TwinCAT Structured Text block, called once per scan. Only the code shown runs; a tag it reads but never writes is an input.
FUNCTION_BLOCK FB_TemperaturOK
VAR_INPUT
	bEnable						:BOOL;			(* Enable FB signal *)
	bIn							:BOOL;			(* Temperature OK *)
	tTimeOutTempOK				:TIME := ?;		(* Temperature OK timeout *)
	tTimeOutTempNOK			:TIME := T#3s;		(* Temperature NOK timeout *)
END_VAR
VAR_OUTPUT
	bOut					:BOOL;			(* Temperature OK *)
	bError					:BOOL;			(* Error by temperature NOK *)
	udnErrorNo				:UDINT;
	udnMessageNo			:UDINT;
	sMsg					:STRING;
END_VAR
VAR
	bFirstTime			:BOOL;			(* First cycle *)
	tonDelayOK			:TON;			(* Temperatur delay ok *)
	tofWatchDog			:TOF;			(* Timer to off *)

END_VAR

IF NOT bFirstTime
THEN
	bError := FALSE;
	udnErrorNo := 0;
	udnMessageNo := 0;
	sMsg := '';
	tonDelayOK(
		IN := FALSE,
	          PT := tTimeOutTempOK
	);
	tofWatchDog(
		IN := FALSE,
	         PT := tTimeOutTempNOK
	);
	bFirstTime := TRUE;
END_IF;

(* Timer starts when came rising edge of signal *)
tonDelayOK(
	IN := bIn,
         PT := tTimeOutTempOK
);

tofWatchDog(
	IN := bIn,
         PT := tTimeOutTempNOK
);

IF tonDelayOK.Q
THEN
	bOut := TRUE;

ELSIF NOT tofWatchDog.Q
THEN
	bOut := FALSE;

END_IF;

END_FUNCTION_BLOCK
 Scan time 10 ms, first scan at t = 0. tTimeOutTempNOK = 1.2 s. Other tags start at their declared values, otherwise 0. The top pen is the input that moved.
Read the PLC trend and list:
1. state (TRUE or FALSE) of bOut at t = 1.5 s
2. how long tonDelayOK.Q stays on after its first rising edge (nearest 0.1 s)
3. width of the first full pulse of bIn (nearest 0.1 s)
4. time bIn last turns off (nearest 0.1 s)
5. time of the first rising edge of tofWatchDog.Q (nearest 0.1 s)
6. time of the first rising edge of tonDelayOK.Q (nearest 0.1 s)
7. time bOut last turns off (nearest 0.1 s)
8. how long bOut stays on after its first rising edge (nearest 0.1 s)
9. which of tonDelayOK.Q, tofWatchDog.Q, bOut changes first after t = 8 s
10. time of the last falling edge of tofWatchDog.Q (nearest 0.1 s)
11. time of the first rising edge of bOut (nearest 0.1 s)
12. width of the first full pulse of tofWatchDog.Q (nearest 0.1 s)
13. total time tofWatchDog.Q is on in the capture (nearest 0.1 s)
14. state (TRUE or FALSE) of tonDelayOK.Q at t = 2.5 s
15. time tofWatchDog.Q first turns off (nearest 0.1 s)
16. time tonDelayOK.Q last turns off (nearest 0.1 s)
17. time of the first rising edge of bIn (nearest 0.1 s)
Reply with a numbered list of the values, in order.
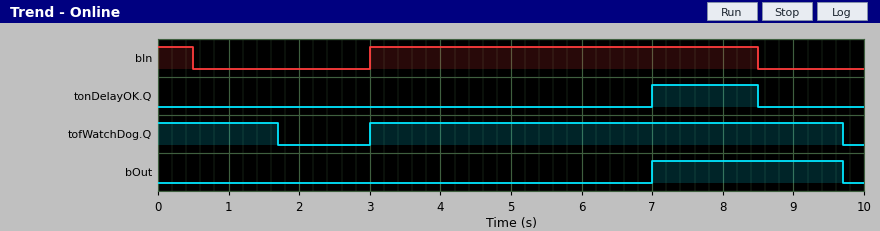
1. FALSE
2. 1.5 s
3. 5.5 s
4. 8.5 s
5. 3.0 s
6. 7.0 s
7. 9.7 s
8. 2.7 s
9. tonDelayOK.Q
10. 9.7 s
11. 7.0 s
12. 6.7 s
13. 8.4 s
14. FALSE
15. 1.7 s
16. 8.5 s
17. 3.0 s
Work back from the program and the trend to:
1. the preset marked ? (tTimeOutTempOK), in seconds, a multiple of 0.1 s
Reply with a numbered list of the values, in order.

1. 4.0 s
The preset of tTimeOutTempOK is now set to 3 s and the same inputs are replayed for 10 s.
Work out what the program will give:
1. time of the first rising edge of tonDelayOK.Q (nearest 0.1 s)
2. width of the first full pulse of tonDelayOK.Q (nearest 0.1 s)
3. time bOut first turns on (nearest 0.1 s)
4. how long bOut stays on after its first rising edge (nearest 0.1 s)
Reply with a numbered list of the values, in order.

1. 6.0 s
2. 2.5 s
3. 6.0 s
4. 3.7 s
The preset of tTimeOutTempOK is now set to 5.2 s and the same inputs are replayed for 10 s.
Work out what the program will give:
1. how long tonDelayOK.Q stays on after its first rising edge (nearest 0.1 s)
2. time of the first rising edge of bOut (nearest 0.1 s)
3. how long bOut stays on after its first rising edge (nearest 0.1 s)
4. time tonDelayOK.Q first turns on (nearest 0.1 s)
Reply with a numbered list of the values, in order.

1. 0.3 s
2. 8.2 s
3. 1.5 s
4. 8.2 s
